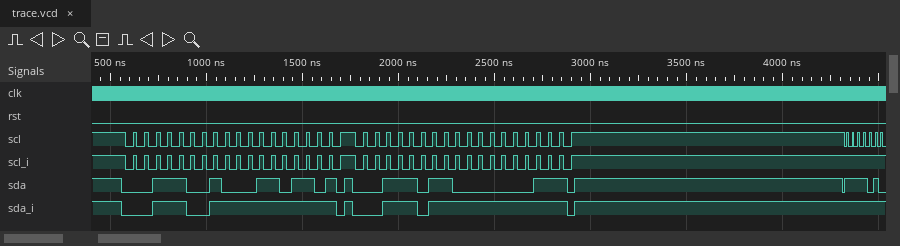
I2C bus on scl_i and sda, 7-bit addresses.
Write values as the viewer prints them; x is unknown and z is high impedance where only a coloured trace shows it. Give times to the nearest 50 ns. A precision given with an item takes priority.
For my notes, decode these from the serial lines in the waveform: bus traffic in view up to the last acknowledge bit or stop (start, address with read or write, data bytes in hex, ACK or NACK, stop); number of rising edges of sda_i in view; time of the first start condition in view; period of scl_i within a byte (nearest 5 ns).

start, address 1C read ACK, 36 NACK, stop, start, address 1D read ACK, 03 NACK, stop
6
550 ns
60 ns
